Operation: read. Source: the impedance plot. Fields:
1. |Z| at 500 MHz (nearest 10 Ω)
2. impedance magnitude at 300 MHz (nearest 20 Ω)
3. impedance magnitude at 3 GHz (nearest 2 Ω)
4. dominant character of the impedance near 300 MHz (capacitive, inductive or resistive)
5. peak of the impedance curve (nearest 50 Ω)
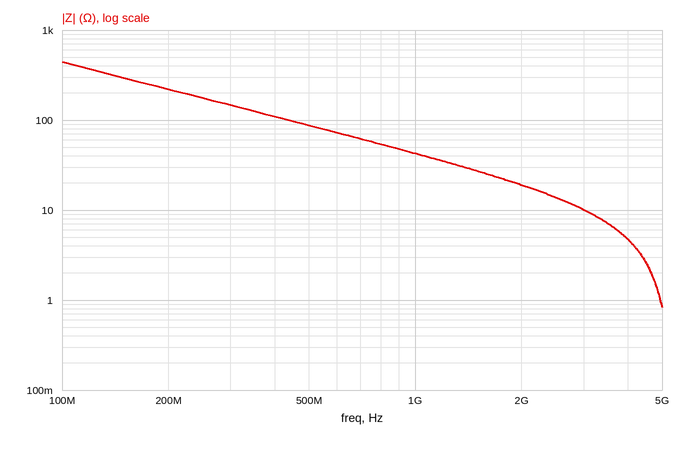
90 Ω
140 Ω
10 Ω
capacitive
450 Ω
